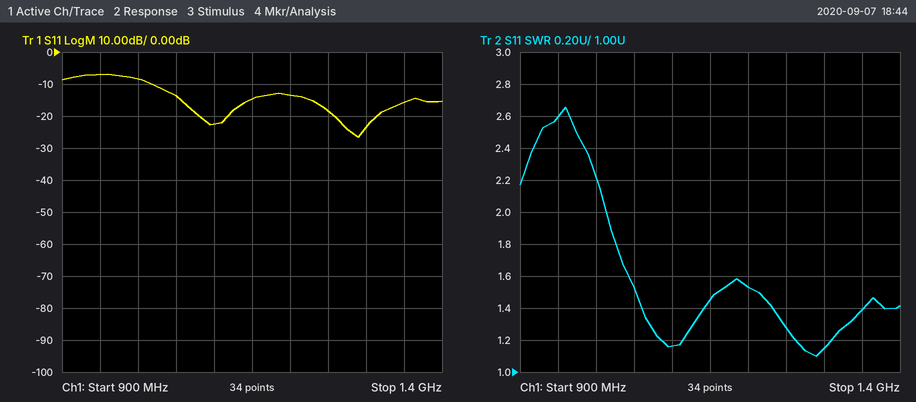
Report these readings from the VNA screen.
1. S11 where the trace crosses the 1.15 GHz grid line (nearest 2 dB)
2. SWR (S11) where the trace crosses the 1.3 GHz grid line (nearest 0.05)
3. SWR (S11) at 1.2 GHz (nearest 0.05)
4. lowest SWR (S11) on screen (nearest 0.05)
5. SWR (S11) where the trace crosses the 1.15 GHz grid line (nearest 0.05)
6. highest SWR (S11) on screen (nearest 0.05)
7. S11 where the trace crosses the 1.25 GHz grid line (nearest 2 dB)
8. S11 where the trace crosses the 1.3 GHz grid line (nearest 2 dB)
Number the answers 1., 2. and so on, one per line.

1. -14 dB
2. 1.15
3. 1.55
4. 1.10
5. 1.45
6. 2.65
7. -18 dB
8. -24 dB
